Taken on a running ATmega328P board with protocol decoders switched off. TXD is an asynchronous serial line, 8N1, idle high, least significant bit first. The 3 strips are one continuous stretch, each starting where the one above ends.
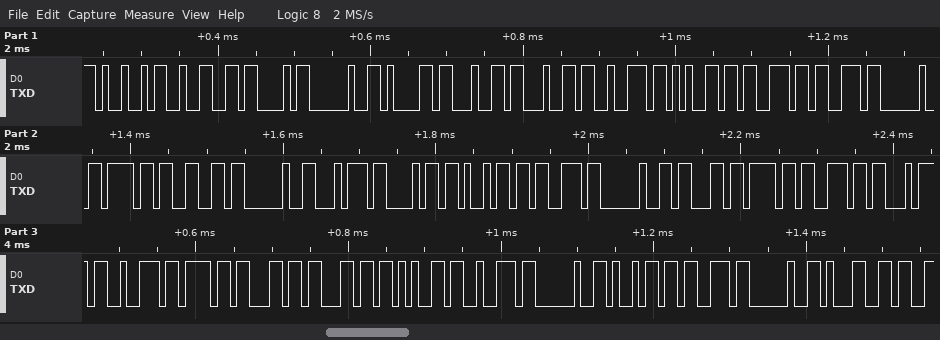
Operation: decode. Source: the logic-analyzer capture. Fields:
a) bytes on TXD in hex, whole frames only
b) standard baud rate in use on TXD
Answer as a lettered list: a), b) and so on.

a) 49 32 43 20 61 64 64 72 65 73 73 20 6F 66 20 74 68 69 73 20 63 6F 6E 74 72 6F 6C 6C 65 72 20 69 73 20 31
b) 115200 baud
